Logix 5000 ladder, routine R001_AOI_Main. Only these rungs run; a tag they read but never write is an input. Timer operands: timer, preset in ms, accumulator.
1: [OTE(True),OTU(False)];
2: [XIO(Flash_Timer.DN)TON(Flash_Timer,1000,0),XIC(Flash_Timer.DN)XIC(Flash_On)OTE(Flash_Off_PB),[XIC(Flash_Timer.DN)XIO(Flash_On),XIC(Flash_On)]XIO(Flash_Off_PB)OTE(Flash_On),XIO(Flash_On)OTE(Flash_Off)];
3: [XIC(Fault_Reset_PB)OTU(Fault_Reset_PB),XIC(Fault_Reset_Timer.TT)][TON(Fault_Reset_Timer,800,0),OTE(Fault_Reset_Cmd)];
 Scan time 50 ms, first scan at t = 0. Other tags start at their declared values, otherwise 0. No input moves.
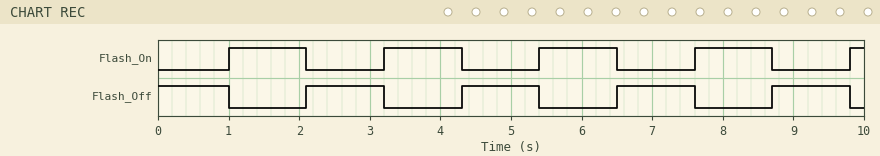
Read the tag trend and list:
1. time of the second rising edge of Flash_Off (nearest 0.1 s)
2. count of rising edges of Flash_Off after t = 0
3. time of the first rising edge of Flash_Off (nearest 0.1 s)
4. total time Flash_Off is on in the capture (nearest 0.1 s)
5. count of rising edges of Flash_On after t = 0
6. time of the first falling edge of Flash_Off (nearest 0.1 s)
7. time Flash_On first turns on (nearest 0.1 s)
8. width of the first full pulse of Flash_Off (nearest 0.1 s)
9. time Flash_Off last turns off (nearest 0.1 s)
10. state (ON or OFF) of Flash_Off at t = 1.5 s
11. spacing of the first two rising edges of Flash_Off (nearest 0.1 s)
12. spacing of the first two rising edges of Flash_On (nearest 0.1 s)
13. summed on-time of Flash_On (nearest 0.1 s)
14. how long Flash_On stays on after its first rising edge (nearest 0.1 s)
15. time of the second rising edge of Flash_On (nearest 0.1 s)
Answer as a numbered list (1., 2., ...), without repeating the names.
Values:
1. 4.3 s
2. 4
3. 2.1 s
4. 5.4 s
5. 5
6. 1.0 s
7. 1.0 s
8. 1.1 s
9. 9.8 s
10. OFF
11. 2.2 s
12. 2.2 s
13. 4.6 s
14. 1.1 s
15. 3.2 s
